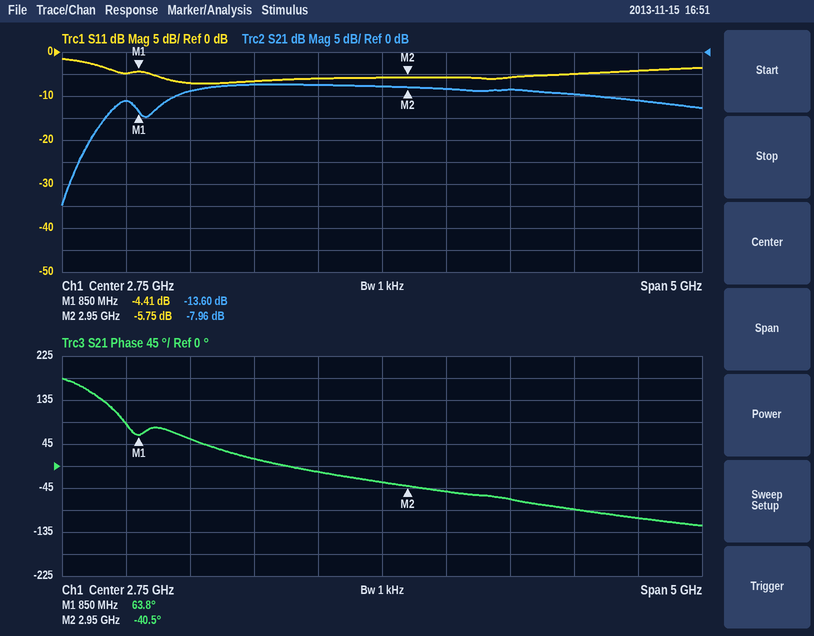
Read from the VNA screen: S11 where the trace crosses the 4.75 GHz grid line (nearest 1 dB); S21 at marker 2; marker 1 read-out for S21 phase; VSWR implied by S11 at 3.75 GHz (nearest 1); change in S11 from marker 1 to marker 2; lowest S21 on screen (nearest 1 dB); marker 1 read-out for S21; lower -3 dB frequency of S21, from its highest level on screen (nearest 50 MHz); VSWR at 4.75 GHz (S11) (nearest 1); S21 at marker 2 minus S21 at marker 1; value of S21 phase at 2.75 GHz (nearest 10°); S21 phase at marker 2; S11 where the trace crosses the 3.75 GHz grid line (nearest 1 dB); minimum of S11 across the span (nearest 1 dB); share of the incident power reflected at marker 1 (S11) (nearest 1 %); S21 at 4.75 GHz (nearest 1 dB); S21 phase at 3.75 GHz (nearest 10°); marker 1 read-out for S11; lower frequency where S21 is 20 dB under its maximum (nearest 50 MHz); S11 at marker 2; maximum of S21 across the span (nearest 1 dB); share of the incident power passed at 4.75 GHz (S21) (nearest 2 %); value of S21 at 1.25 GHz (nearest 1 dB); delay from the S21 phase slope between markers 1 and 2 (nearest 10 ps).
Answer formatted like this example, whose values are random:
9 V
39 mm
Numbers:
-4 dB
-7.96 dB
63.8°
3
-1.34 dB
-35 dB
-13.60 dB
1.10 GHz
4
5.64 dB
-30°
-40.5°
-6 dB
-7 dB
36 %
-11 dB
-70°
-4.41 dB
350 MHz
-5.75 dB
-7 dB
8 %
-9 dB
140 ps
